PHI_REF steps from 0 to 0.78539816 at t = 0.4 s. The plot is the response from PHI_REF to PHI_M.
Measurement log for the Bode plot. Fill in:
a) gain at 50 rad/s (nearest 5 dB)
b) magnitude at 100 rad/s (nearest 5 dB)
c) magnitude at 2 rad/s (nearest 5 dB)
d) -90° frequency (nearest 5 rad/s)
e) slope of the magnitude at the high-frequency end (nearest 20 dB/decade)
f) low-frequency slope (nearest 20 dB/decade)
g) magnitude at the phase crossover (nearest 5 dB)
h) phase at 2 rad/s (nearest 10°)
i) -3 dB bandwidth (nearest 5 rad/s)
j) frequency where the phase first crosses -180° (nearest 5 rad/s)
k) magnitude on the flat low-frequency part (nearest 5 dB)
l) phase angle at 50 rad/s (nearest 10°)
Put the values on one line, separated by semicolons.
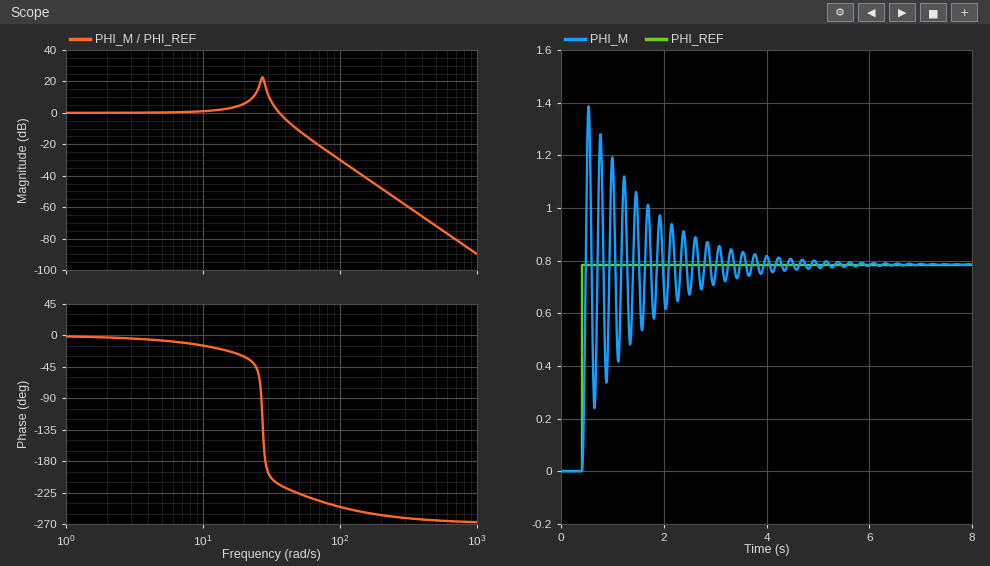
-10 dB; -30 dB; 0 dB; 25 rad/s; -60 dB/decade; 0 dB/decade; 15 dB; 0°; 40 rad/s; 30 rad/s; 0 dB; -230°
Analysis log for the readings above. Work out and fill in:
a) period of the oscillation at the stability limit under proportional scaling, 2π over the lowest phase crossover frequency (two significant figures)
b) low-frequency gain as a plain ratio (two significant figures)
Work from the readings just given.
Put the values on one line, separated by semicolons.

0.21 s; 1.0
